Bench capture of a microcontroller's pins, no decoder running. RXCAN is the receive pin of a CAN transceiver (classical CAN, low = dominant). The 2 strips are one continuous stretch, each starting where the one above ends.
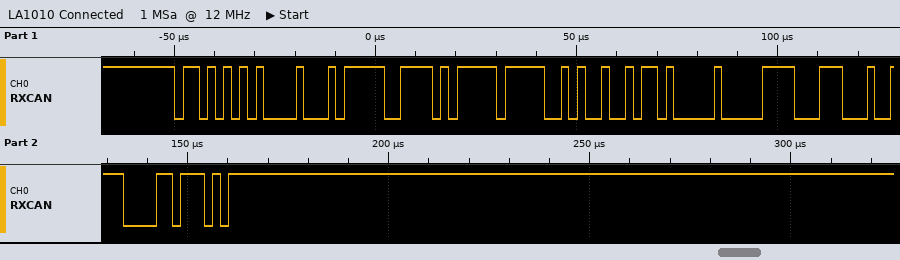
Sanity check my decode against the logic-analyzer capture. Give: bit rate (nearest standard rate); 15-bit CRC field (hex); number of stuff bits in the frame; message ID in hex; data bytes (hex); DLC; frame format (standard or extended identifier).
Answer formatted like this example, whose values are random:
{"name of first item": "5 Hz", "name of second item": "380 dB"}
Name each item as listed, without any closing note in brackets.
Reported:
{"bit rate": "500 kbit/s", "15-bit CRC field": "0x386E", "number of stuff bits in the frame": "5", "message ID in hex": "0x6AA", "data bytes": "BE F5 FF A9 2D 00 38 E2", "DLC": "8", "frame format": "standard"}
